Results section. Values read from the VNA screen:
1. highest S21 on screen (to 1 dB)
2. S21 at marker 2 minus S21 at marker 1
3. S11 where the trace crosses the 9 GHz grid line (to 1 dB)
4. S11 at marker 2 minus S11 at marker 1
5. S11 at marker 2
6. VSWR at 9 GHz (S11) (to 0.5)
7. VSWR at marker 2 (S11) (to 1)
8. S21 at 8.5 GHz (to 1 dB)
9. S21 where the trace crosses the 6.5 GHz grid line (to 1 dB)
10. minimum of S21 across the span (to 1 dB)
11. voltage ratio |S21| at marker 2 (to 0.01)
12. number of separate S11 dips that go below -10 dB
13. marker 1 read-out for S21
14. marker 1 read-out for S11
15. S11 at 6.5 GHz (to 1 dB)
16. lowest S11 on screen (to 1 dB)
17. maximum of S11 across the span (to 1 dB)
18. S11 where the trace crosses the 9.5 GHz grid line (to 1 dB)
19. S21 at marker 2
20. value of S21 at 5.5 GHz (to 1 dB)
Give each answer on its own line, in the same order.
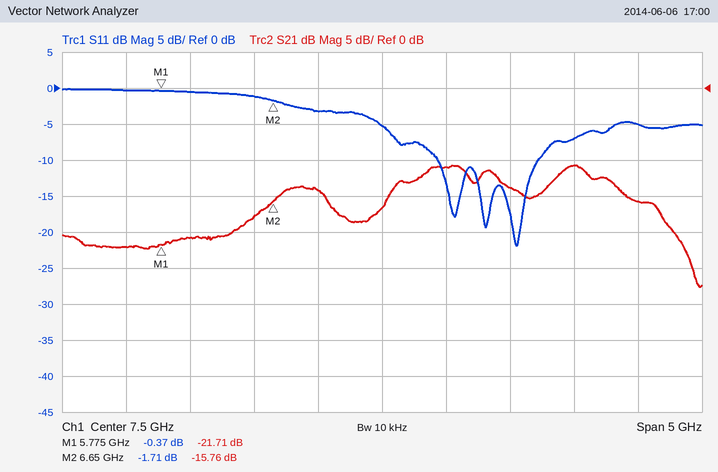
-11 dB
5.95 dB
-7 dB
-1.34 dB
-1.71 dB
2.5
10
-14 dB
-18 dB
-28 dB
0.16
3
-21.71 dB
-0.37 dB
-1 dB
-22 dB
0 dB
-5 dB
-15.76 dB
-22 dB
